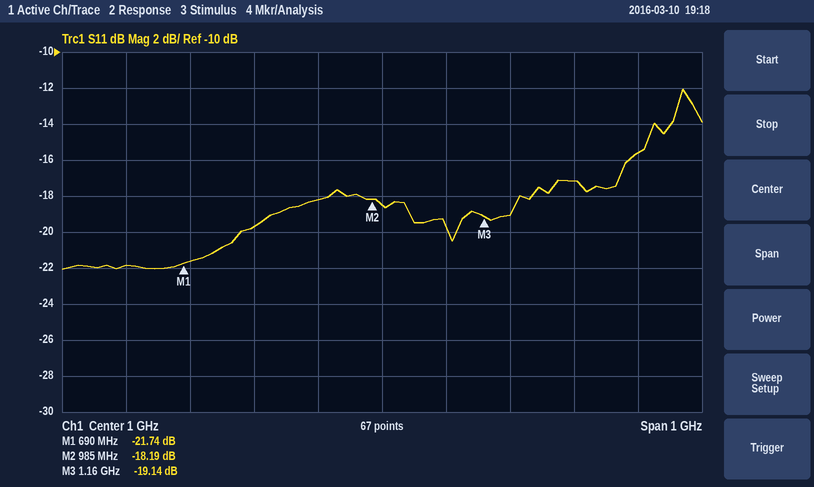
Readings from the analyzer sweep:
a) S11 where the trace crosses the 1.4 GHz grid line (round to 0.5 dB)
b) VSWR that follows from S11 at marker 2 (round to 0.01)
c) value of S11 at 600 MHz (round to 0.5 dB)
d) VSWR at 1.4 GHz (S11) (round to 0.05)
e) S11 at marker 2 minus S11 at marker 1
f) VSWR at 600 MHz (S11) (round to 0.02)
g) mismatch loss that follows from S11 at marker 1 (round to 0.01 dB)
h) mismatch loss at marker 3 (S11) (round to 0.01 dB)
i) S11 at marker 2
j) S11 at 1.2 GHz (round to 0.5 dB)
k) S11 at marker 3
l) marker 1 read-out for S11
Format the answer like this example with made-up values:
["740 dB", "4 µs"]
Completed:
["-15.5 dB", "1.28", "-22.0 dB", "1.40", "3.55 dB", "1.18", "0.03 dB", "0.05 dB", "-18.19 dB", "-19.0 dB", "-19.14 dB", "-21.74 dB"]
